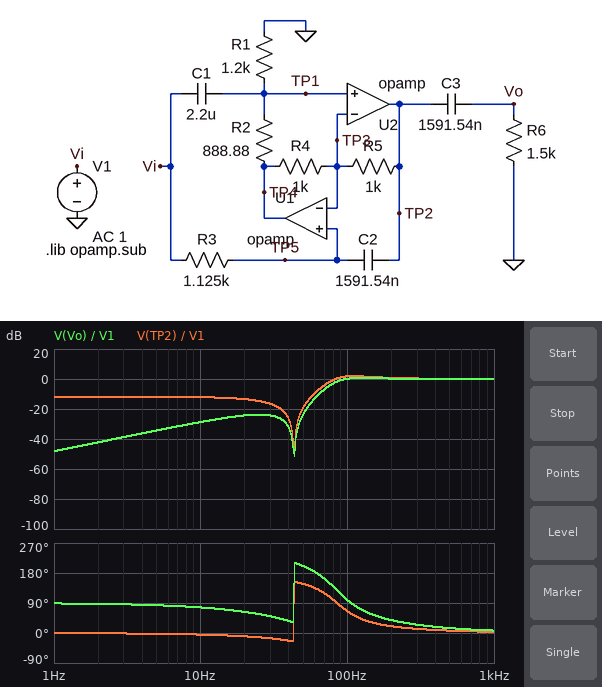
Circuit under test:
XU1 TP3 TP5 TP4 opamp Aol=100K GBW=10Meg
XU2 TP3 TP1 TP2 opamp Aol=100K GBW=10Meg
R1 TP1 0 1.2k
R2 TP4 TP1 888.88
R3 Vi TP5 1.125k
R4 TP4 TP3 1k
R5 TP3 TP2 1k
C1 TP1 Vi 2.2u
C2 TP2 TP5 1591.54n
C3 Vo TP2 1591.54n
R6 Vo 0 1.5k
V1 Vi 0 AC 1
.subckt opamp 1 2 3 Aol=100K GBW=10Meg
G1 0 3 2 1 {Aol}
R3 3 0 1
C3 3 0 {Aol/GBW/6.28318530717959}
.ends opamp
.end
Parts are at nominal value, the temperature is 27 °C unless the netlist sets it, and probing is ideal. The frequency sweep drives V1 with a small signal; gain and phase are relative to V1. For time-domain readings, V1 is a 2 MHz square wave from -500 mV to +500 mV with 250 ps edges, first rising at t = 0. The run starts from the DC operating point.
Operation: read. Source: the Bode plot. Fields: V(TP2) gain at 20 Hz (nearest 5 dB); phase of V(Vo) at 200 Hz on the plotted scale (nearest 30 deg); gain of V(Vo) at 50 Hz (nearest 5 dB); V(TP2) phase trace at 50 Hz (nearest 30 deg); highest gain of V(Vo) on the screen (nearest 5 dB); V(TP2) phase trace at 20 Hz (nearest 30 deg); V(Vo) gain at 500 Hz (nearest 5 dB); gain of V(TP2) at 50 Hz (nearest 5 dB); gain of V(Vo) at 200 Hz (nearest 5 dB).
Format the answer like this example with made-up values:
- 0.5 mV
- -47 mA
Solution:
- -15 dB
- 30 deg
- -25 dB
- 150 deg
- 0 dB
- 0 deg
- 0 dB
- -20 dB
- 0 dB
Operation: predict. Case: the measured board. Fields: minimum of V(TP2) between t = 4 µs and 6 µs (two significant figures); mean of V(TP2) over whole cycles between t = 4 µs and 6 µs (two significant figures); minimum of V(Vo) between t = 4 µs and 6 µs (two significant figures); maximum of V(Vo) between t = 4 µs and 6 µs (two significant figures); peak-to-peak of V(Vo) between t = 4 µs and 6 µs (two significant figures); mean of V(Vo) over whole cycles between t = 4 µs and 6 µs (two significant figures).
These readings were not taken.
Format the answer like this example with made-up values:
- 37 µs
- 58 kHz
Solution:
- -340 mV
- 370 mV
- -210 mV
- 1.2 V
- 1.4 V
- 500 mV
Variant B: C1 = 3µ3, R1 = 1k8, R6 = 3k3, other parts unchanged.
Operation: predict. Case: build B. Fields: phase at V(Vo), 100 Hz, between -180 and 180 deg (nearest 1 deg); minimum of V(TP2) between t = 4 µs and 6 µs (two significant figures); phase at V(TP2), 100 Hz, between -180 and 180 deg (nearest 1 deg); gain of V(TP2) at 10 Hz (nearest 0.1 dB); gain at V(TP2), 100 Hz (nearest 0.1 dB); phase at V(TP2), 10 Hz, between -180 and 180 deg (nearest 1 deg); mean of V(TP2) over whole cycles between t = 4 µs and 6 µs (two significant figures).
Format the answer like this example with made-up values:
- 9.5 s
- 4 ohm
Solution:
- 44 deg
- -460 mV
- 27 deg
- -6.1 dB
- 2.3 dB
- -3 deg
- 250 mV
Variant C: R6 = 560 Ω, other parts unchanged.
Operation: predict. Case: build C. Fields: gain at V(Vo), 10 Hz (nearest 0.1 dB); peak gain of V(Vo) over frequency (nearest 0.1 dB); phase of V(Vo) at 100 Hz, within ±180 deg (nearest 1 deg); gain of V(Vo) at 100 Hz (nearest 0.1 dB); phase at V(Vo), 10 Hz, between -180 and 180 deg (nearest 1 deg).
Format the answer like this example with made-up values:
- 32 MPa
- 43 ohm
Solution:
- -37.2 dB
- 0 dB
- 126 deg
- -4.5 dB
- 82 deg
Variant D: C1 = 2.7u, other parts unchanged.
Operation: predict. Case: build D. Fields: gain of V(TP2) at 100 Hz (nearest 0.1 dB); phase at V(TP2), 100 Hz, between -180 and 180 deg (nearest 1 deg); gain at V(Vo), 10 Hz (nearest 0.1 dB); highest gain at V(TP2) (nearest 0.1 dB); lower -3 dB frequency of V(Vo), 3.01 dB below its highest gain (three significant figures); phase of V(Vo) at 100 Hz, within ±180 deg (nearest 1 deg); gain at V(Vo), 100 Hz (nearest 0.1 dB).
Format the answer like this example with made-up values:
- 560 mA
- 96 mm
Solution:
- 2.4 dB
- 50 deg
- -28.8 dB
- 2.5 dB
- 73.2 Hz
- 84 deg
- 0.8 dB
